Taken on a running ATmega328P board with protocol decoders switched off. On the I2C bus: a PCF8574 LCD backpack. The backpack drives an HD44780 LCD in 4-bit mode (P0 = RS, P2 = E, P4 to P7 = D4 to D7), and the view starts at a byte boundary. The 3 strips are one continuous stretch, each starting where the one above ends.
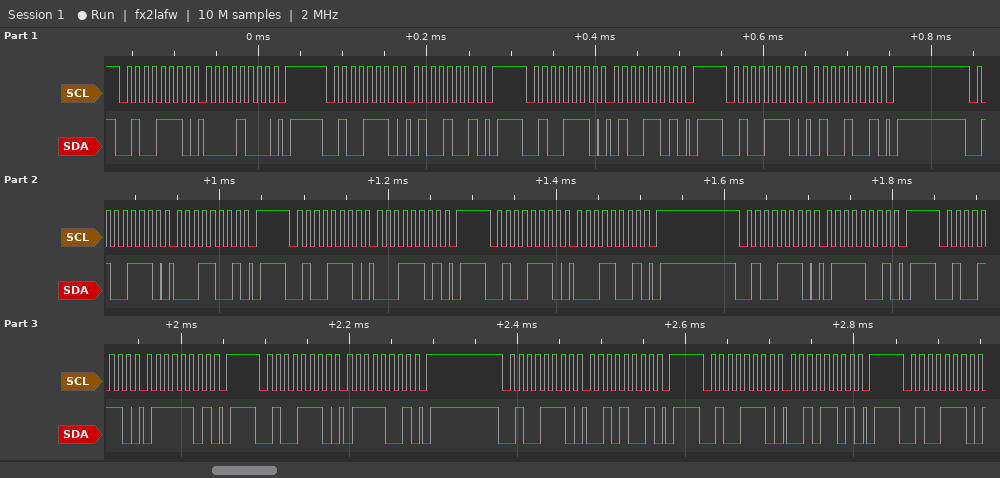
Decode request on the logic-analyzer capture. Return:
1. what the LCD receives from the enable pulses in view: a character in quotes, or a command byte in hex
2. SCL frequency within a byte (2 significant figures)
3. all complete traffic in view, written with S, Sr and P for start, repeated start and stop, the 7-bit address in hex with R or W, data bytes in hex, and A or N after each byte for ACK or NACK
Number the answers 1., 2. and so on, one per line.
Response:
1. 'A'
2. 100 kHz
3. S 27W A 08 A P S 27W A 49 A P S 27W A 4D A P S 27W A 49 A P S 27W A 19 A P S 27W A 1D A P S 27W A 19 A P S 27W A 79 A P S 27W A 7D A P S 27W A 79 A P S 27W A 29 A P S 27W A 2D A P S 27W A
